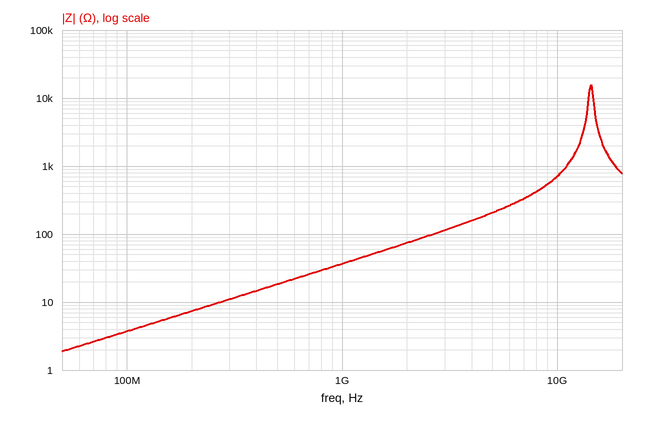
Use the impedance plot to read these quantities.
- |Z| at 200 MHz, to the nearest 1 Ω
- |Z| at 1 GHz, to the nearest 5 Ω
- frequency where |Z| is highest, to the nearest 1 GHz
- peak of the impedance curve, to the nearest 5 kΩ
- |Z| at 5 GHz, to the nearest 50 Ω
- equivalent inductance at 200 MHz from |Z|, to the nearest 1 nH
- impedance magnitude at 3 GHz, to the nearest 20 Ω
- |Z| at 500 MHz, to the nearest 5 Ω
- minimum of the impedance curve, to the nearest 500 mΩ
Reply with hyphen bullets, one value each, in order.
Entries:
- 7 Ω
- 35 Ω
- 14 GHz
- 15 kΩ
- 200 Ω
- 6 nH
- 120 Ω
- 20 Ω
- 2.0 Ω
